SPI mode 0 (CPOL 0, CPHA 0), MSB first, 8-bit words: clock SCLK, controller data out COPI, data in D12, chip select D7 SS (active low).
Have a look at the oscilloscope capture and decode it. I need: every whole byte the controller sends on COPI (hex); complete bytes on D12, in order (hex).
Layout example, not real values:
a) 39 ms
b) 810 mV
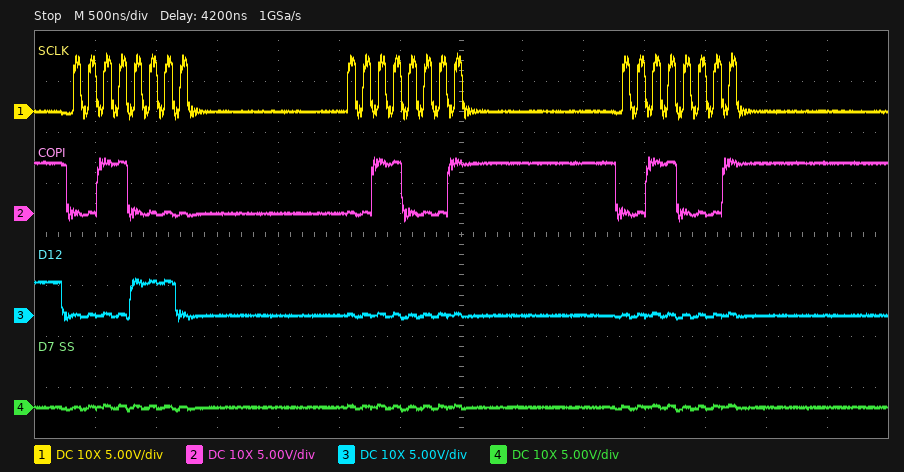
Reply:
a) 30 31 31
b) 0E 00 00
